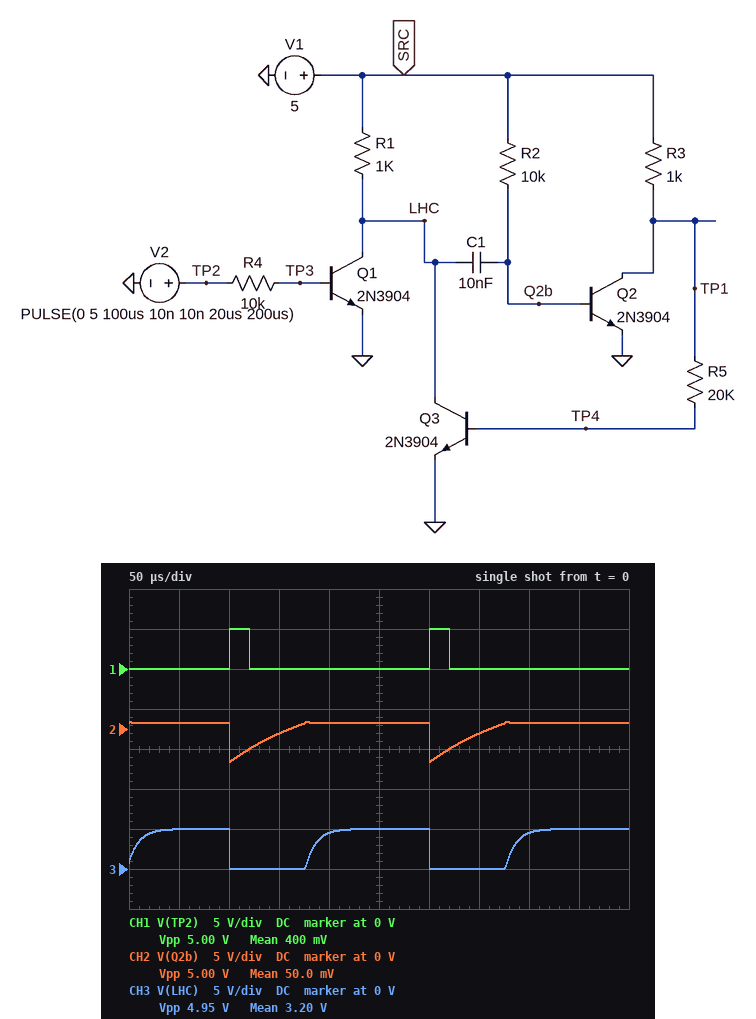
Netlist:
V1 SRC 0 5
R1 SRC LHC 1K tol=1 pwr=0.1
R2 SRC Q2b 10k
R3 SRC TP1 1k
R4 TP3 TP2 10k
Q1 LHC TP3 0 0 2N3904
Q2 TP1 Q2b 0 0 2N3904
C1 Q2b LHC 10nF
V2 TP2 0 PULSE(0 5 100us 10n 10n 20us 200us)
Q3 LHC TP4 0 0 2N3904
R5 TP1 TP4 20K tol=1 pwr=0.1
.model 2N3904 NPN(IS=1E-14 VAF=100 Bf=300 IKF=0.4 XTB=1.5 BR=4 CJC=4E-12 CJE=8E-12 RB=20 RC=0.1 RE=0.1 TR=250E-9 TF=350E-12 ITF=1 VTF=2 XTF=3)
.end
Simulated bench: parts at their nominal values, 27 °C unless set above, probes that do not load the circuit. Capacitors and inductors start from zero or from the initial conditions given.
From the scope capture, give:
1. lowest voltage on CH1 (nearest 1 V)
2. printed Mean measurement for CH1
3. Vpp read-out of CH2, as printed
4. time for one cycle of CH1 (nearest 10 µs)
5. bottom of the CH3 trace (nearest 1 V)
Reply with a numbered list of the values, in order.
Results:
1. 0 V
2. 400 mV
3. 5.00 V
4. 200 µs
5. 0 V
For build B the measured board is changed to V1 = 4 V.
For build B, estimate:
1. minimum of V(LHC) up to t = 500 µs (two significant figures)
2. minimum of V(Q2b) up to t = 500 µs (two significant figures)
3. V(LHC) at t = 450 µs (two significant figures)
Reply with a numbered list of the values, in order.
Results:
1. 30 mV
2. -3.2 V
3. 4.0 V
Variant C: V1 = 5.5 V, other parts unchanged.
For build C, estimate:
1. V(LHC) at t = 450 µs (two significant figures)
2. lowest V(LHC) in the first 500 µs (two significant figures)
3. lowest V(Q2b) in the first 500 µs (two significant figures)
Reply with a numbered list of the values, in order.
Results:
1. 5.5 V
2. 34 mV
3. -4.6 V
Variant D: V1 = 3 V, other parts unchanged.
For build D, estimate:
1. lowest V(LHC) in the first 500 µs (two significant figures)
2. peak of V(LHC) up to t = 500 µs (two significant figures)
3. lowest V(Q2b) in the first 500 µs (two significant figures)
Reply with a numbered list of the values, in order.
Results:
1. 26 mV
2. 3.0 V
3. -2.2 V
